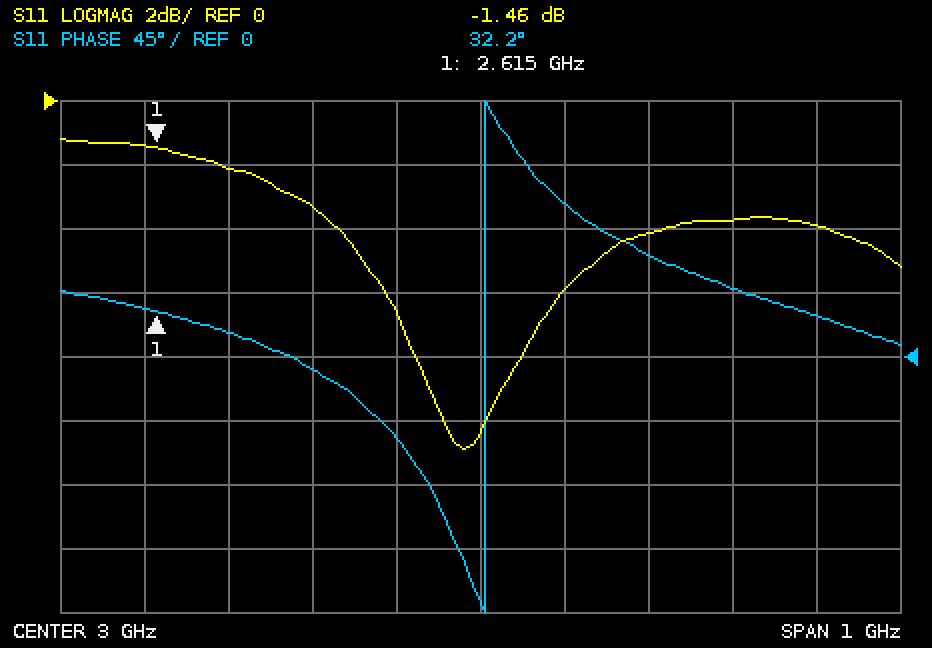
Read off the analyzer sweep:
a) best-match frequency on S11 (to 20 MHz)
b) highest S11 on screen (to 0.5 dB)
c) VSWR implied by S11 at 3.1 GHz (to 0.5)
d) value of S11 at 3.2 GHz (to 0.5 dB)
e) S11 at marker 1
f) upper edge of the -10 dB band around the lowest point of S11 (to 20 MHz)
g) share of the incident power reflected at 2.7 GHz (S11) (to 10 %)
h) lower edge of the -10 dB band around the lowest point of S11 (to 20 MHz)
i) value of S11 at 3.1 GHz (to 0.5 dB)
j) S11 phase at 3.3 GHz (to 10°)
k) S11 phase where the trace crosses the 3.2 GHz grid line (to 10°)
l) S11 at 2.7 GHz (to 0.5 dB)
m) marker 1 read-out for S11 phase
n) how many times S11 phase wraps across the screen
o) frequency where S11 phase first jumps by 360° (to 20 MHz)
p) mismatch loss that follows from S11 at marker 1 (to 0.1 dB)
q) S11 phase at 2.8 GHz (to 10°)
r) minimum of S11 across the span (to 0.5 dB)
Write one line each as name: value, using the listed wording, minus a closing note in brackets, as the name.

best-match frequency on S11: 2.98 GHz
highest S11 on screen: -1.0 dB
VSWR implied by S11 at 3.1 GHz: 3.0
value of S11 at 3.2 GHz: -4.0 dB
S11 at marker 1: -1.46 dB
upper edge of the -10 dB band around the lowest point of S11: 3.00 GHz
share of the incident power reflected at 2.7 GHz (S11): 60 %
lower edge of the -10 dB band around the lowest point of S11: 2.96 GHz
value of S11 at 3.1 GHz: -6.0 dB
S11 phase at 3.3 GHz: 50°
S11 phase where the trace crosses the 3.2 GHz grid line: 70°
S11 at 2.7 GHz: -2.0 dB
marker 1 read-out for S11 phase: 32.2°
how many times S11 phase wraps across the screen: 1
frequency where S11 phase first jumps by 360°: 3.00 GHz
mismatch loss that follows from S11 at marker 1: 5.4 dB
S11 phase at 2.8 GHz: -10°
minimum of S11 across the span: -11.0 dB
